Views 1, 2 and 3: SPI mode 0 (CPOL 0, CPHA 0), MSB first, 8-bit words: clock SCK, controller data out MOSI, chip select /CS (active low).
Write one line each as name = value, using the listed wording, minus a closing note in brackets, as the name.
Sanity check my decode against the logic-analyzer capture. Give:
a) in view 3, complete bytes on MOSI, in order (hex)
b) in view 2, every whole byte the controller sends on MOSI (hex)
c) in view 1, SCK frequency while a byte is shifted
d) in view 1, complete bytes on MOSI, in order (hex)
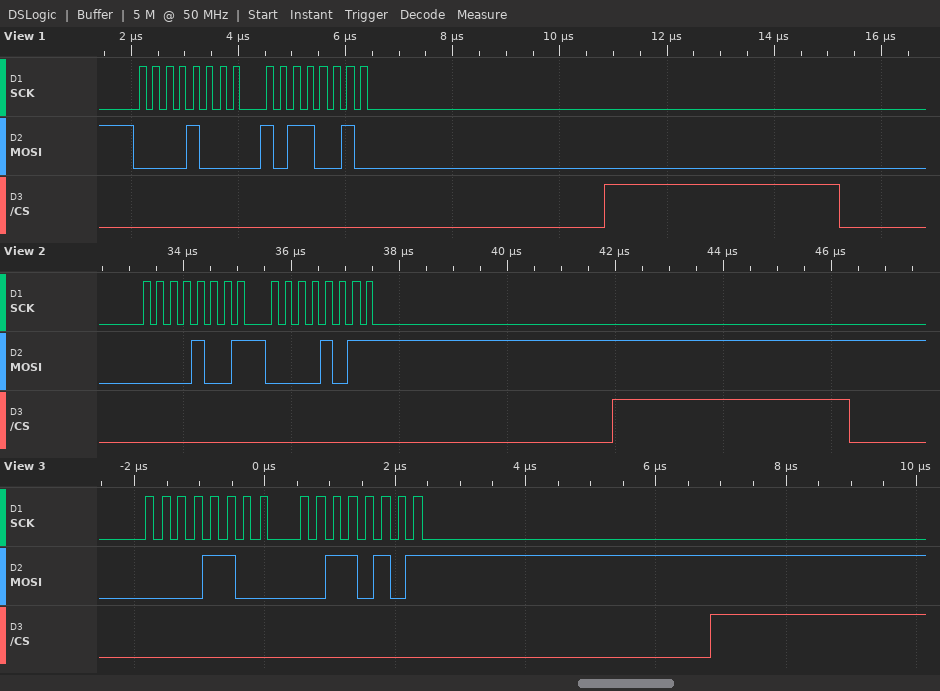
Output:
in view 3, complete bytes on MOSI, in order = 0x0C 0x35
in view 2, every whole byte the controller sends on MOSI = 09 0B
in view 1, SCK frequency while a byte is shifted = 4 MHz
in view 1, complete bytes on MOSI, in order = 0x08 0xB2
